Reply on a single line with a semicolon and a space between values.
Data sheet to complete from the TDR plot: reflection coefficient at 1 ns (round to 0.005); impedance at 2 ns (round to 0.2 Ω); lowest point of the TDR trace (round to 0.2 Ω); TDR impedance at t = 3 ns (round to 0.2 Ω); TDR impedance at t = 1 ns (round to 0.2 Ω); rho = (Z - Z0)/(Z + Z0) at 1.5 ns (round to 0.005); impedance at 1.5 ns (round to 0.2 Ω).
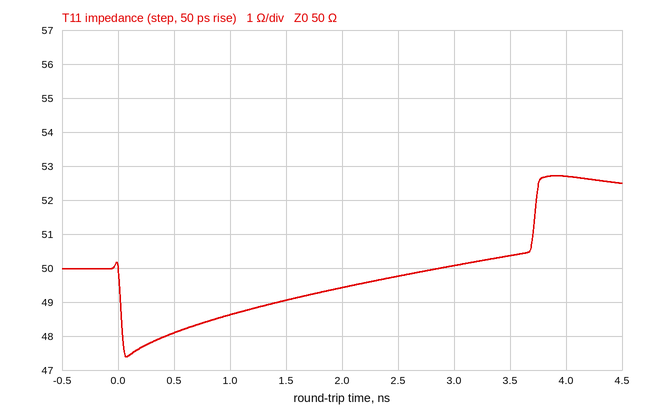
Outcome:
-0.015; 49.4 Ω; 47.4 Ω; 50.0 Ω; 48.6 Ω; -0.010; 49.0 Ω
